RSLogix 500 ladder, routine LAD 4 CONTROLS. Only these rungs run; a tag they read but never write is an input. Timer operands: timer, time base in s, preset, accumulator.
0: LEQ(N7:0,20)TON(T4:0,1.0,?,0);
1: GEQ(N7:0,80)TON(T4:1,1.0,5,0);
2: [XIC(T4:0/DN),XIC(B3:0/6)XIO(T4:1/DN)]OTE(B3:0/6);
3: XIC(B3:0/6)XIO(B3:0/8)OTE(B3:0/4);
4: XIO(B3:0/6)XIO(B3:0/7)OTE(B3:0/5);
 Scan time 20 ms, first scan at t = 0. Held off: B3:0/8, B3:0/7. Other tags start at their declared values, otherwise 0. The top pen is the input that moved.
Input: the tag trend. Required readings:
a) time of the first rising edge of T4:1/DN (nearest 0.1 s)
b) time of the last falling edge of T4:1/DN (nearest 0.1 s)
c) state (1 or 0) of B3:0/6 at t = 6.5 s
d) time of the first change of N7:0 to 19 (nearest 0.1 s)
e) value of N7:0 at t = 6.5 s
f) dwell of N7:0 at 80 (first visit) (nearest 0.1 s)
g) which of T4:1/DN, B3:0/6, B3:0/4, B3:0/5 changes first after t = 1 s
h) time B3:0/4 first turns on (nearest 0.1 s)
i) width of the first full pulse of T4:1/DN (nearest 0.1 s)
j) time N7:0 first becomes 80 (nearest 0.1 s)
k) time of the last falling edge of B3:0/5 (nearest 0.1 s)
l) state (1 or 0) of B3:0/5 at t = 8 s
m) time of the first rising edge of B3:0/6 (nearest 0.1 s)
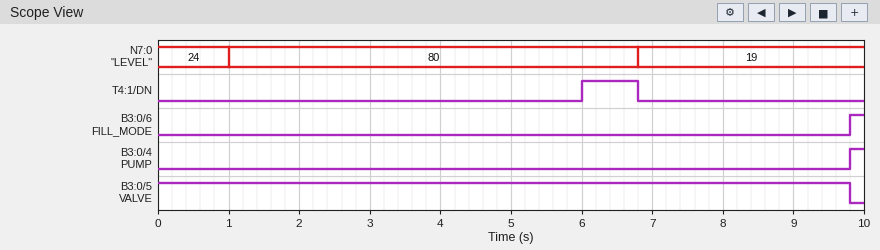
6.0 s
6.8 s
0
6.8 s
80
5.8 s
T4:1/DN
9.8 s
0.8 s
1.0 s
9.8 s
1
9.8 s
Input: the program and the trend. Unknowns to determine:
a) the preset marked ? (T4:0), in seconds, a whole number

3 s
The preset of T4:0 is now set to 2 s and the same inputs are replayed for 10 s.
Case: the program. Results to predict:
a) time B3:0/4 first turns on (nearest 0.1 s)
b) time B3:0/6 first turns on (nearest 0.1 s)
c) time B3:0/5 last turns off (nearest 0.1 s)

8.8 s
8.8 s
8.8 s
